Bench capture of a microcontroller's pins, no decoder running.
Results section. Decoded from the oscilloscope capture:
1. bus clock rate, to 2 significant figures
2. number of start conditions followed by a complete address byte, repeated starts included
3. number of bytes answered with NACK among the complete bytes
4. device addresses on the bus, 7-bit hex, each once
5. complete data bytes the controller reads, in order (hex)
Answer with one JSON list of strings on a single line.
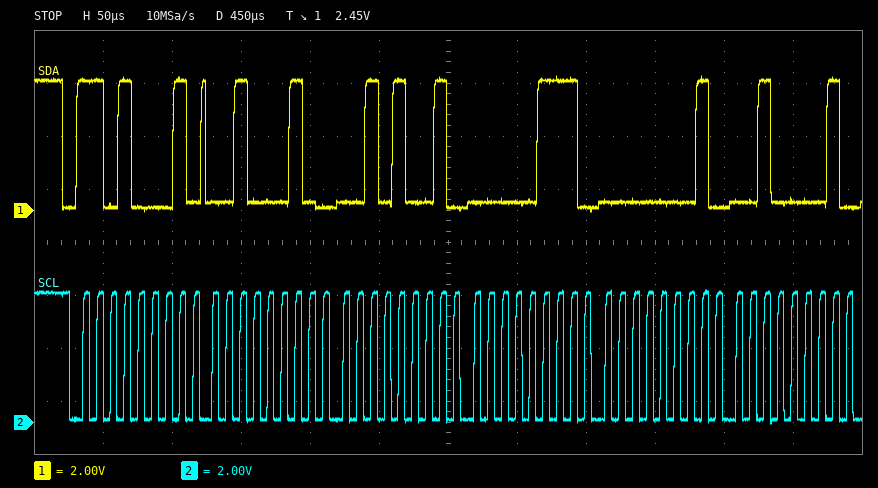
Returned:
["100 kHz", "1", "0", "0x68", "22 29 07 01 21"]
